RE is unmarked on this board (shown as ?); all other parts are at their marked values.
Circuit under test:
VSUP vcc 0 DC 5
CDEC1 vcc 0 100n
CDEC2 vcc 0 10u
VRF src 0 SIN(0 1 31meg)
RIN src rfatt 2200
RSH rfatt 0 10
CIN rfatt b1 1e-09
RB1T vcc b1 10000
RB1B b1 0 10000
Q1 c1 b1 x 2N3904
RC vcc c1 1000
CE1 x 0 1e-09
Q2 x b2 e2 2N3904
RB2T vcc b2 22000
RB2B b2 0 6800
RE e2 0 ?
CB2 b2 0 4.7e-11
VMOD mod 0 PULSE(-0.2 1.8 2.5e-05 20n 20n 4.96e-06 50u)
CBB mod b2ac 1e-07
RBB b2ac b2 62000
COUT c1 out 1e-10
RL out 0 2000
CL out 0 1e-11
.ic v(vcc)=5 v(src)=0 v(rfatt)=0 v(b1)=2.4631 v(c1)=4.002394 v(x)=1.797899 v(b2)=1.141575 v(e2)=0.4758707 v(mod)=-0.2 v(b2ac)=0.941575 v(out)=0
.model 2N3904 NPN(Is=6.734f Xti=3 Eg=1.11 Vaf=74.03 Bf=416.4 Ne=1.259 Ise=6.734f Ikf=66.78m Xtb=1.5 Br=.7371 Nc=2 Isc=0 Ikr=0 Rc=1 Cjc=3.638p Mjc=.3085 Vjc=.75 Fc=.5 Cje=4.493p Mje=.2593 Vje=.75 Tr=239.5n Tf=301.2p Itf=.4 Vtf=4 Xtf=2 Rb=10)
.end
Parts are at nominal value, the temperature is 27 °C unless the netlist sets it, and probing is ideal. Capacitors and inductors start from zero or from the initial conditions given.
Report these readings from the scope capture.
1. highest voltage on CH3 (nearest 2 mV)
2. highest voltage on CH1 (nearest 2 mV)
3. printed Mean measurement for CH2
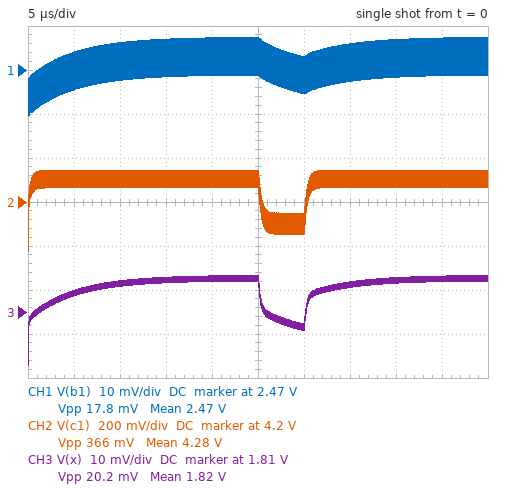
1.818 V
2.478 V
4.28 V
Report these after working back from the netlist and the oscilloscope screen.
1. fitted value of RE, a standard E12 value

680 Ω
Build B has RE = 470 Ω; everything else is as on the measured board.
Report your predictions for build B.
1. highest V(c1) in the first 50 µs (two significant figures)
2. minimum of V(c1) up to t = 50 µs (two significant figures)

4.1 V
3.7 V
